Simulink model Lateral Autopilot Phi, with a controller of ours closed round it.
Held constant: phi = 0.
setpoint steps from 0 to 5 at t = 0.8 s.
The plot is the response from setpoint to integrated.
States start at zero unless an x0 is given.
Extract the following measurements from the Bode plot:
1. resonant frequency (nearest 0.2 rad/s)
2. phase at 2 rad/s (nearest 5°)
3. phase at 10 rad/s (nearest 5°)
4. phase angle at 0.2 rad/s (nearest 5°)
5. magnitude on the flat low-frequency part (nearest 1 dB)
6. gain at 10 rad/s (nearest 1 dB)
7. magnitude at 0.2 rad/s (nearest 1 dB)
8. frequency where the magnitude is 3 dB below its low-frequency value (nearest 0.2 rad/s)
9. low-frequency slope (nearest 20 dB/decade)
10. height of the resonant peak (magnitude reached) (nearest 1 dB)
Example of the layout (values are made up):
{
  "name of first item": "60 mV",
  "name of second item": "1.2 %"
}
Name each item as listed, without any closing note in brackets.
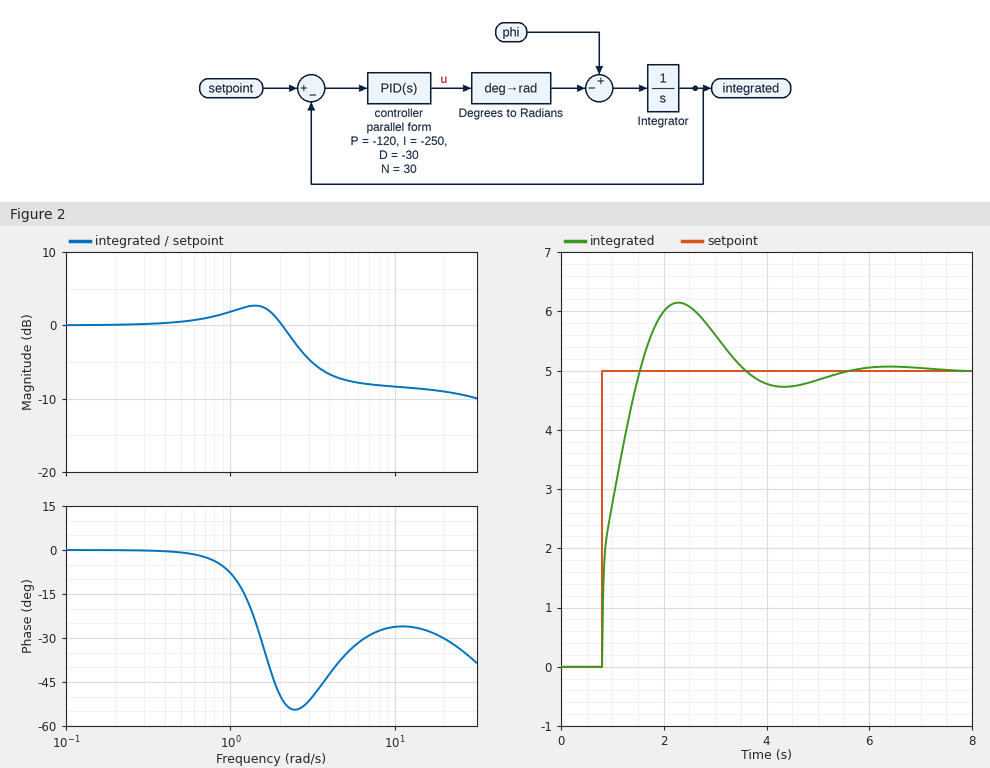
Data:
{
  "resonant frequency": "1.4 rad/s",
  "phase at 2 rad/s": "-50°",
  "phase at 10 rad/s": "-25°",
  "phase angle at 0.2 rad/s": "0°",
  "magnitude on the flat low-frequency part": "0 dB",
  "gain at 10 rad/s": "-8 dB",
  "magnitude at 0.2 rad/s": "0 dB",
  "frequency where the magnitude is 3 dB below its low-frequency value": "2.6 rad/s",
  "low-frequency slope": "0 dB/decade",
  "height of the resonant peak (magnitude reached)": "3 dB"
}
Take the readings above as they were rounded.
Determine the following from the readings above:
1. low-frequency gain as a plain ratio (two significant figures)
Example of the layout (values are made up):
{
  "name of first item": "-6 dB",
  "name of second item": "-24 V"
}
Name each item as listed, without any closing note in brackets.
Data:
{
  "low-frequency gain as a plain ratio": "1.0"
}
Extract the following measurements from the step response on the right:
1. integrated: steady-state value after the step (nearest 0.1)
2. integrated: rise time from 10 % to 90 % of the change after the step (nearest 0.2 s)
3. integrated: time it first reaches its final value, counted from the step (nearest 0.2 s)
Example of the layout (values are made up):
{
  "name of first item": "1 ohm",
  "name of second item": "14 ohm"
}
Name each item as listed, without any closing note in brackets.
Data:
{
  "integrated: steady-state value after the step": "5.0",
  "integrated: rise time from 10 % to 90 % of the change after the step": "0.6 s",
  "integrated: time it first reaches its final value, counted from the step": "0.8 s"
}
